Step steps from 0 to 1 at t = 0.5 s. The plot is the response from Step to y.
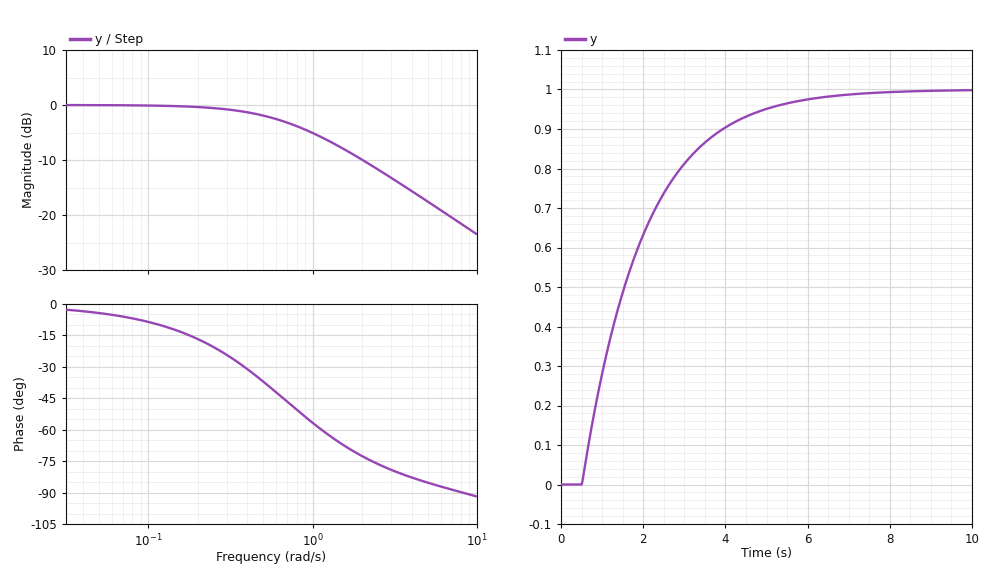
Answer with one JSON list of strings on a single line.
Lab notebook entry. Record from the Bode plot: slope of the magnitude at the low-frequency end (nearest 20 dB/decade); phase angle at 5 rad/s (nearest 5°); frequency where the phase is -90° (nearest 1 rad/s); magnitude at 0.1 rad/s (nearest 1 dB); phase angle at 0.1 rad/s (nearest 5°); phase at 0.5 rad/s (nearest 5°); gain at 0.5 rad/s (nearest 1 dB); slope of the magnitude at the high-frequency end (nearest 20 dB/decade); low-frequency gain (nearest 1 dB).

["0 dB/decade", "-85°", "8 rad/s", "0 dB", "-10°", "-35°", "-2 dB", "-20 dB/decade", "0 dB"]
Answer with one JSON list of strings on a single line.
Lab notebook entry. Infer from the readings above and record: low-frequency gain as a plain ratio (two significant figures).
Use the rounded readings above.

["1.0"]
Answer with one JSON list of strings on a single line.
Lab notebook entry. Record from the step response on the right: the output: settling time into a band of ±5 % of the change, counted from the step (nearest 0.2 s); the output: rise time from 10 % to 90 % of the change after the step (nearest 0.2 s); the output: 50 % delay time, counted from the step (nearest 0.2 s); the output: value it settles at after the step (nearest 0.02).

["4.4 s", "3.2 s", "1.0 s", "1.00"]
